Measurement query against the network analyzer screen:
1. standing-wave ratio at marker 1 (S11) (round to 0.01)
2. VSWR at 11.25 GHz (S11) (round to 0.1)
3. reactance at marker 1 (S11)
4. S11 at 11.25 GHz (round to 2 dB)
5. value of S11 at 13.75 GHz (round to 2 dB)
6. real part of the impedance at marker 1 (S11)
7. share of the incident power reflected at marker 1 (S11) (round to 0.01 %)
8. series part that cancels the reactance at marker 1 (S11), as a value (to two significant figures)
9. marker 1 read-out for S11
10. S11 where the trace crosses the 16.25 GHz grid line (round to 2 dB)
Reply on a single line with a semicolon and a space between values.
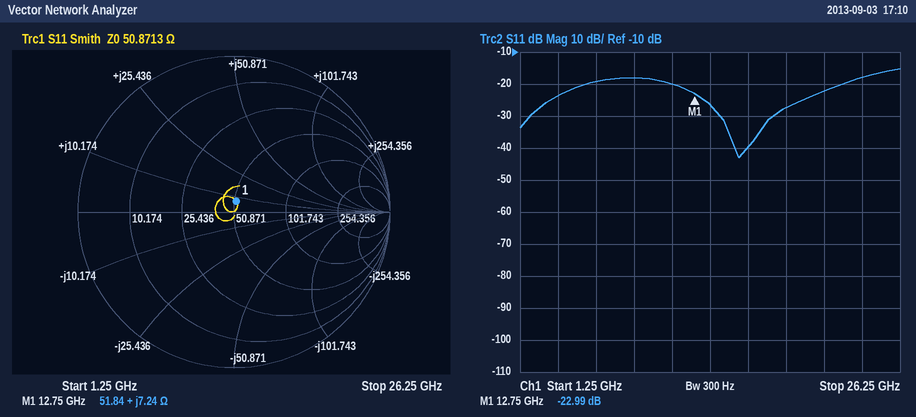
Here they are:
1.15; 1.2; +7.24 Ω; -20 dB; -26 dB; 51.84 Ω; 0.50 %; 1.7 pF; -22.99 dB; -40 dB
